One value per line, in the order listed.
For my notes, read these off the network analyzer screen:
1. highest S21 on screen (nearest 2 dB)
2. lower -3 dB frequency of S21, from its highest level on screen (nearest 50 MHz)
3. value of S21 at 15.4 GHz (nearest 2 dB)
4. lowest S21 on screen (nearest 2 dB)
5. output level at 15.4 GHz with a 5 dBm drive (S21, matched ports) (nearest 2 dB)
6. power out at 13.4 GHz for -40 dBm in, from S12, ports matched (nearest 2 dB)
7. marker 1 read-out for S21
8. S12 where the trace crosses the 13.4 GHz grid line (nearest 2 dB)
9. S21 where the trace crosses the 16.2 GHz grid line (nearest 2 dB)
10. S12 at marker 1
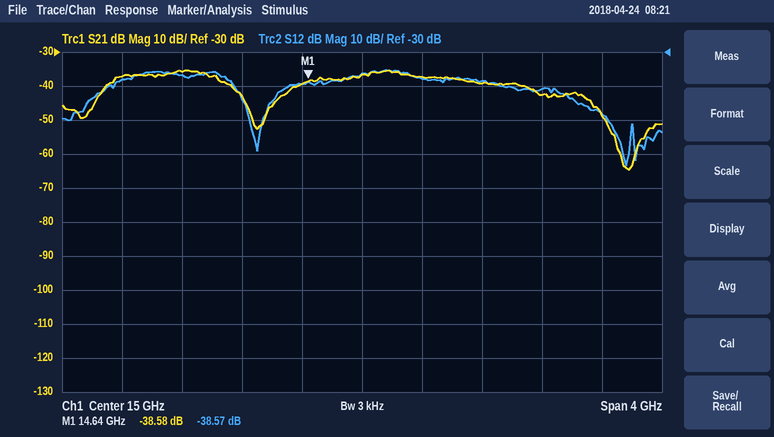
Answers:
-36 dB
13.35 GHz
-38 dB
-64 dB
-32 dBm
-78 dBm
-38.58 dB
-38 dB
-42 dB
-38.57 dB
